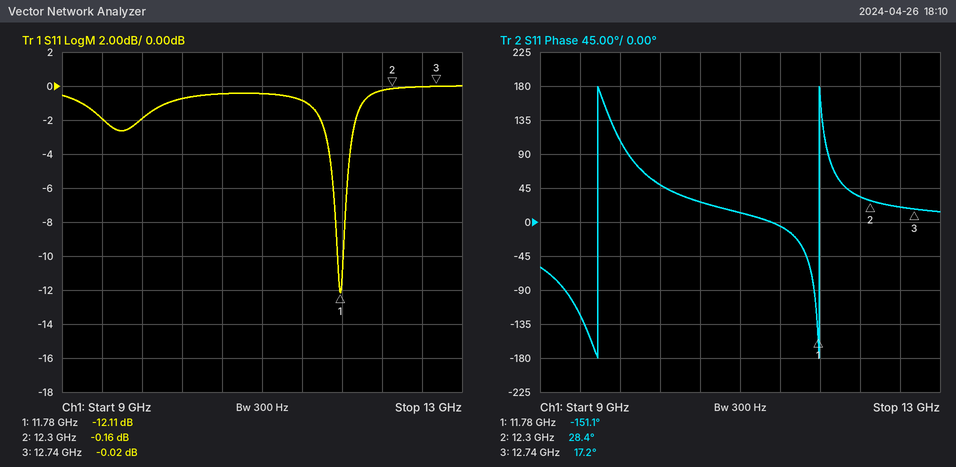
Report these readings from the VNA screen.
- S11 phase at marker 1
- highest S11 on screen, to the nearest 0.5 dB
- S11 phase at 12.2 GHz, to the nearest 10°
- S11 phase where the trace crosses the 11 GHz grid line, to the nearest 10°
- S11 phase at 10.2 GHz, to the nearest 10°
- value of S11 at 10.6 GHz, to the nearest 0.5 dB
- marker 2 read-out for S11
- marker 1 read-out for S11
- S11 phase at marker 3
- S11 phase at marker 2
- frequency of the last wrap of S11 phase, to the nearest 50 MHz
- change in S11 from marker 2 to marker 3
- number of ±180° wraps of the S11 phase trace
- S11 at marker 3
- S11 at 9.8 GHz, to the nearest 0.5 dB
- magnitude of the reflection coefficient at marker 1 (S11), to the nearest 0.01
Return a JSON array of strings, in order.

["-151.1°", "0.0 dB", "30°", "10°", "50°", "-0.5 dB", "-0.16 dB", "-12.11 dB", "17.2°", "28.4°", "11.80 GHz", "0.14 dB", "2", "-0.02 dB", "-2.0 dB", "0.25"]
